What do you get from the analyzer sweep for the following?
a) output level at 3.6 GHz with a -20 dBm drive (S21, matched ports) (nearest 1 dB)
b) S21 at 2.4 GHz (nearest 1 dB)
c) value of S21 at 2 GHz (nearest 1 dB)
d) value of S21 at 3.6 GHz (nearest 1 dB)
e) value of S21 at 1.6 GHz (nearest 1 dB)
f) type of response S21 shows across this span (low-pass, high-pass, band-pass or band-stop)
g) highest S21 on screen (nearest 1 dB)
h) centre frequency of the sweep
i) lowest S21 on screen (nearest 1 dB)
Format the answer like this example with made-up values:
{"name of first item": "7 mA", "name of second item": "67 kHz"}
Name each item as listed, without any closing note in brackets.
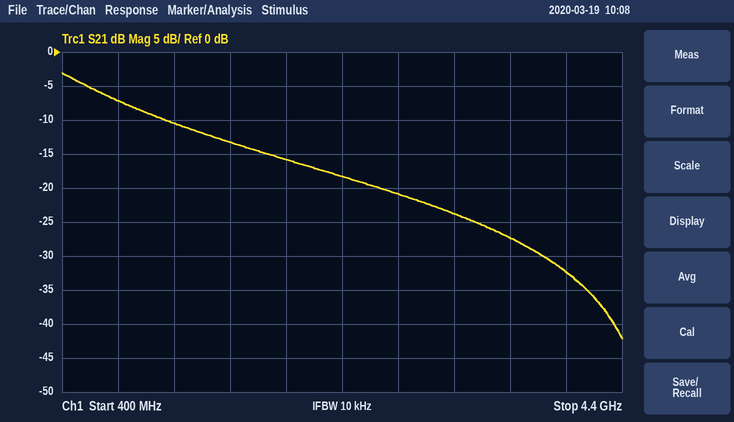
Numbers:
{"output level at 3.6 GHz with a -20 dBm drive (S21, matched ports)": "-47 dBm", "S21 at 2.4 GHz": "-18 dB", "value of S21 at 2 GHz": "-16 dB", "value of S21 at 3.6 GHz": "-27 dB", "value of S21 at 1.6 GHz": "-13 dB", "type of response S21 shows across this span": "low-pass", "highest S21 on screen": "-3 dB", "centre frequency of the sweep": "2.4 GHz", "lowest S21 on screen": "-42 dB"}
